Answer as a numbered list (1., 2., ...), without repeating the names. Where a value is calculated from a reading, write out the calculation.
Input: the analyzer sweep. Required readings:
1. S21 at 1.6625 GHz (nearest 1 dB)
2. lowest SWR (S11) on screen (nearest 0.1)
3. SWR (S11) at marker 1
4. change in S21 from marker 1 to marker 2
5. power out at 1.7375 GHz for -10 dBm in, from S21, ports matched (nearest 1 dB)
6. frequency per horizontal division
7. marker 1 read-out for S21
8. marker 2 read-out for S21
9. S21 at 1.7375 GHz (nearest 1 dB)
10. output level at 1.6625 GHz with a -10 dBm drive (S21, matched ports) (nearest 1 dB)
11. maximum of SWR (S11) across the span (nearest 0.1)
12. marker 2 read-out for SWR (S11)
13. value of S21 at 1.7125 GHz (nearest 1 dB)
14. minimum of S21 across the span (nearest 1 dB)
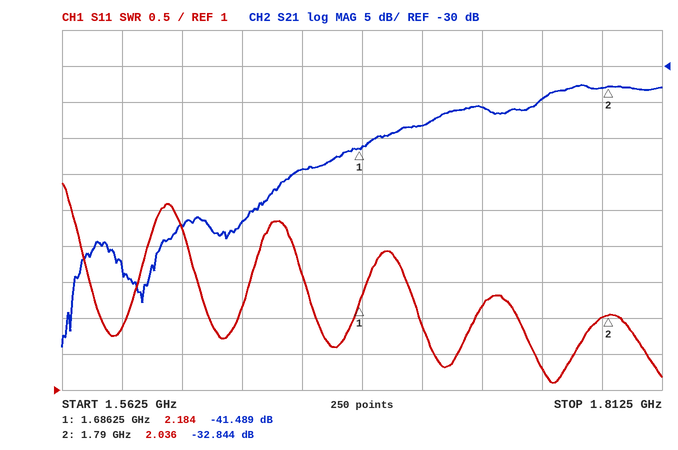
1. -44 dB
2. 1.1
3. 2.184
4. -32.844 − (-41.489) = 8.645 dB
5. -10 dBm + (-36 dB) = -46 dBm
6. 25 MHz
7. -41.489 dB
8. -32.844 dB
9. -36 dB
10. -10 dBm + (-44 dB) = -54 dBm
11. 3.9
12. 2.036
13. -38 dB
14. -69 dB
